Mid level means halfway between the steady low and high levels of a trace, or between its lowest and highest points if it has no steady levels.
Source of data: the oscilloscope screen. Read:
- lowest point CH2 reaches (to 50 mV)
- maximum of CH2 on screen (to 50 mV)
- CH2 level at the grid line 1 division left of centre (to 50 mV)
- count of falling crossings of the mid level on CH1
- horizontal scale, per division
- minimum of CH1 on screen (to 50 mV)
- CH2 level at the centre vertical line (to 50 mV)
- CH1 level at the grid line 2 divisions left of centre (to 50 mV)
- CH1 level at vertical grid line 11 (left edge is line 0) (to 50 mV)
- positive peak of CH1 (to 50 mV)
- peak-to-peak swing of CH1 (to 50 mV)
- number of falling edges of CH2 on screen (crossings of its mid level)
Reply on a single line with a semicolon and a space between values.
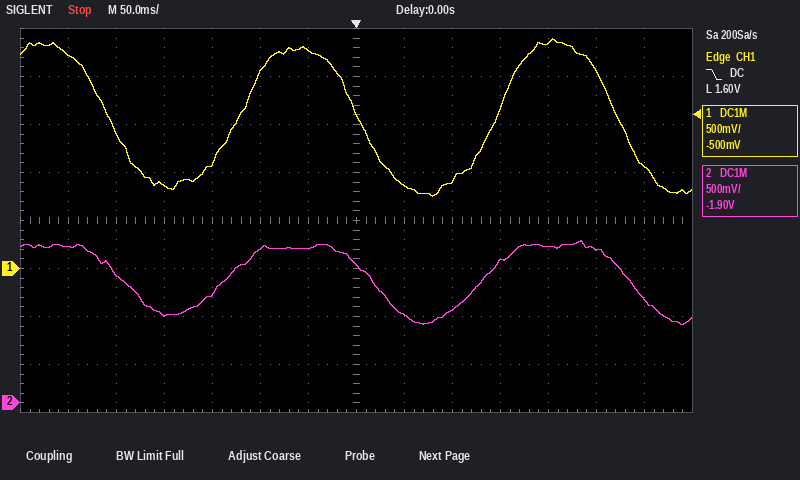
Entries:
800 mV; 1.70 V; 1.60 V; 3; 50 ms; 750 mV; 1.45 V; 2.05 V; 2.35 V; 2.40 V; 1.65 V; 3
